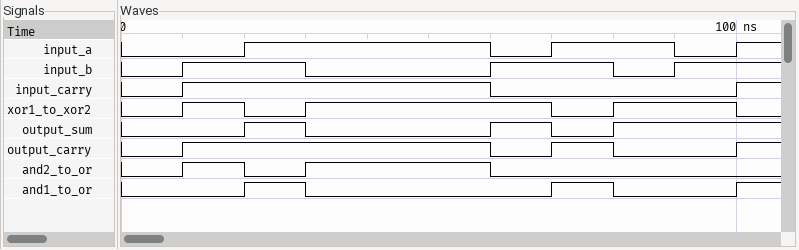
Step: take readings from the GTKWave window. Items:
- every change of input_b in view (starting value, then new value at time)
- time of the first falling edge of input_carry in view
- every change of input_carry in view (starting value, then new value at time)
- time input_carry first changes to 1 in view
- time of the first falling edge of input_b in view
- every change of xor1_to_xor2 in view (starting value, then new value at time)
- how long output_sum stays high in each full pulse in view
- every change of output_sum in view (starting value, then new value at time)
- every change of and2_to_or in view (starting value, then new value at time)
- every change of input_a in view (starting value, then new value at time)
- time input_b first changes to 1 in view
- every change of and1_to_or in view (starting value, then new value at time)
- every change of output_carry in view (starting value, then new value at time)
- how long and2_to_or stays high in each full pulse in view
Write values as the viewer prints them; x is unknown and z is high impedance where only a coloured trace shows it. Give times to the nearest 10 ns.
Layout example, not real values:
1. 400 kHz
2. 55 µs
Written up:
1. 0, 1 at 10 ns, 0 at 30 ns, 1 at 60 ns, 0 at 80 ns, 1 at 90 ns
2. 60 ns
3. 0, 1 at 10 ns, 0 at 60 ns, 1 at 100 ns
4. 10 ns
5. 30 ns
6. 0, 1 at 10 ns, 0 at 20 ns, 1 at 30 ns, 0 at 70 ns, 1 at 80 ns, 0 at 100 ns
7. 10 ns, 10 ns
8. 0, 1 at 20 ns, 0 at 30 ns, 1 at 60 ns, 0 at 70 ns, 1 at 80 ns
9. 0, 1 at 10 ns, 0 at 20 ns, 1 at 30 ns, 0 at 60 ns
10. 0, 1 at 20 ns, 0 at 60 ns, 1 at 70 ns, 0 at 90 ns, 1 at 100 ns
11. 10 ns
12. 0, 1 at 20 ns, 0 at 30 ns, 1 at 70 ns, 0 at 80 ns, 1 at 100 ns
13. 0, 1 at 10 ns, 0 at 60 ns, 1 at 70 ns, 0 at 80 ns, 1 at 100 ns
14. 10 ns, 30 ns
